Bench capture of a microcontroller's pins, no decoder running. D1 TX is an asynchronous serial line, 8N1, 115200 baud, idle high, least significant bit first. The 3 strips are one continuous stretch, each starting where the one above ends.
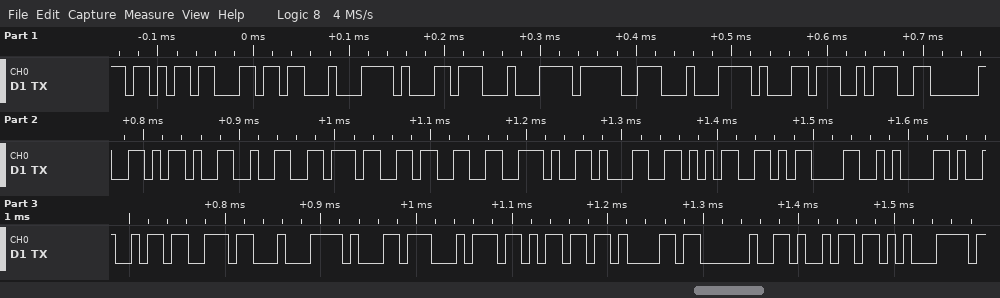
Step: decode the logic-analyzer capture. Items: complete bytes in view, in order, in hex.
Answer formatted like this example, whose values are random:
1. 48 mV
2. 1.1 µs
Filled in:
1. 0x6B 0x6C 0xC4 0xB1 0xC4 0x9F 0xC4 0xB1 0x3A 0x20 0x2D 0x32 0x37 0x33 0x2E 0x31 0x35 0x0D 0x0A 0x49 0x73 0xC4 0xB1 0x74 0x6D 0x61 0x20 0x69 0xC5
